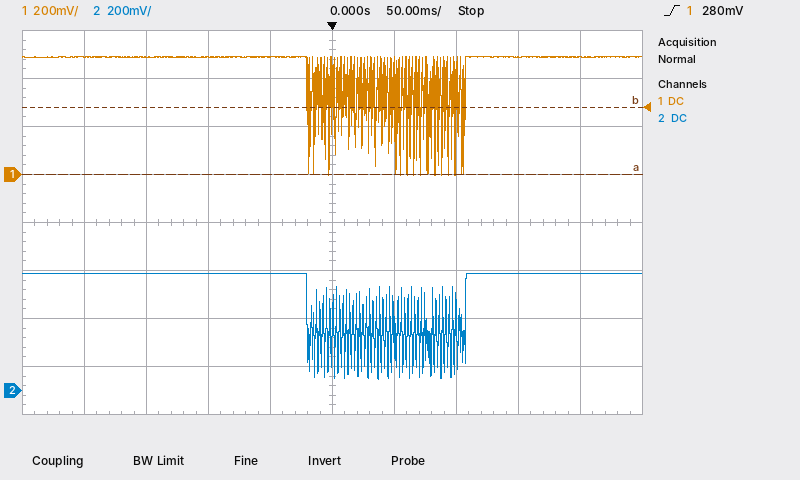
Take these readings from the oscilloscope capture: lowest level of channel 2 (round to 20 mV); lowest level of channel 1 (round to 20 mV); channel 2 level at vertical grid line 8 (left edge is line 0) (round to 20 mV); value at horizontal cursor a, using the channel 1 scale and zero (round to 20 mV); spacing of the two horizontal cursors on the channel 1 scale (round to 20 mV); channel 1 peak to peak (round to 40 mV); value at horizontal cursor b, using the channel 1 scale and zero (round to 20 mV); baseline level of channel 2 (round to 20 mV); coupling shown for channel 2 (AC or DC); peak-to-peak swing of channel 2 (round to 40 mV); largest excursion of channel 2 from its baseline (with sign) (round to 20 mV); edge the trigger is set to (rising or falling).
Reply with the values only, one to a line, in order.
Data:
40 mV
0 mV
480 mV
0 mV
280 mV
480 mV
280 mV
480 mV
DC
440 mV
-440 mV
rising
